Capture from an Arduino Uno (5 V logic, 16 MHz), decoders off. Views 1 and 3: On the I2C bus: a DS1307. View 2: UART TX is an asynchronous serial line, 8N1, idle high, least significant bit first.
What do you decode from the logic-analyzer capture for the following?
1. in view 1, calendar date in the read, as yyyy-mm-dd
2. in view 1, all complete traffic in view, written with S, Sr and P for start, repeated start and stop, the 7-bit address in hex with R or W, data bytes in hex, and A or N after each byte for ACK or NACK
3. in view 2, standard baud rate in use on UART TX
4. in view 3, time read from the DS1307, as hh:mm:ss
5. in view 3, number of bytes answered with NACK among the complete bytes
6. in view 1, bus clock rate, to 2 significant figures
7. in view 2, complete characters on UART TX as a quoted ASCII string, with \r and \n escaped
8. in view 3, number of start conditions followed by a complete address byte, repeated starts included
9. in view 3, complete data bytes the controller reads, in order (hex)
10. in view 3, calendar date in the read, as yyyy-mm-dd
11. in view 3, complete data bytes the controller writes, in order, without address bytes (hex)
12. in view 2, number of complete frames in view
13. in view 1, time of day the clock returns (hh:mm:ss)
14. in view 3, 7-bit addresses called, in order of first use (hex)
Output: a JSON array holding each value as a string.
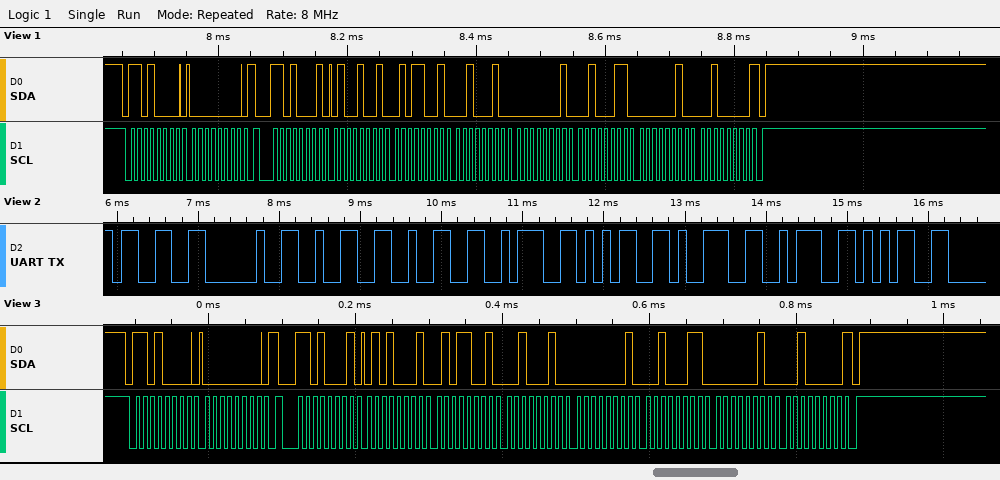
["2020-02-23", "S 68W A 00 A Sr 68R A 49 A 59 A 22 A 01 A 23 A 02 A 20 N P", "9600 baud", "22:59:51", "1", "100 kHz", "\"3 22:59:5\"", "2", "51 59 22 01 23 02 20", "2020-02-23", "00", "9", "22:59:49", "0x68"]
